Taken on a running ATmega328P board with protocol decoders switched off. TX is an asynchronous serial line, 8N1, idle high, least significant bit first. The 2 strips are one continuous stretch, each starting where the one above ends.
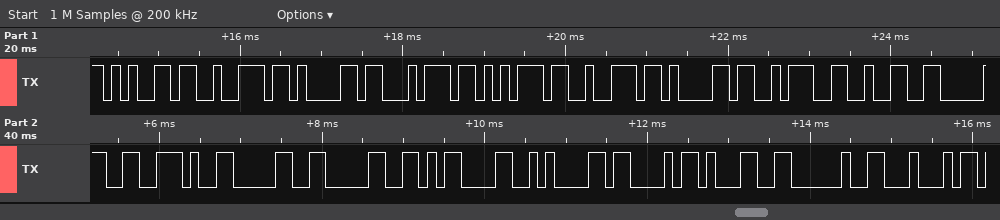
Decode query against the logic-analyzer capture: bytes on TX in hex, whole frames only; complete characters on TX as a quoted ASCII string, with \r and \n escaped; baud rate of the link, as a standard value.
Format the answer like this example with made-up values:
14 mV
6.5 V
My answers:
65 72 61 74 75 72 61 3A 32 30 2E 30 30 0D 0A 43 31 20 44
"eratura:20.00\r\nC1 D"
9600 baud
